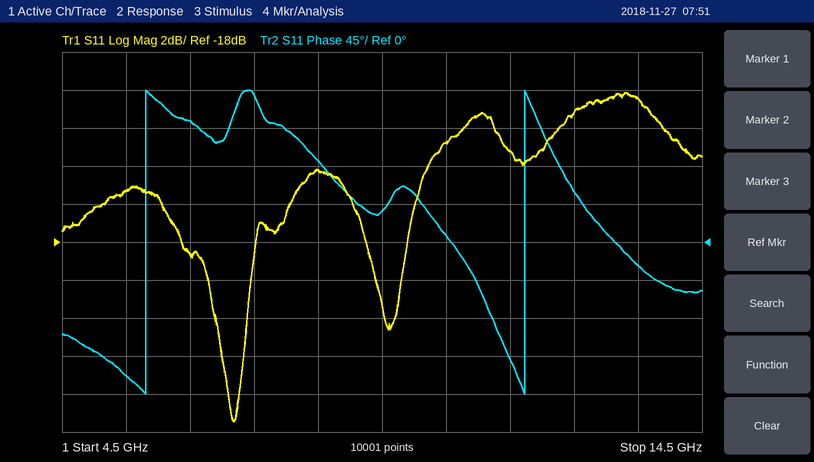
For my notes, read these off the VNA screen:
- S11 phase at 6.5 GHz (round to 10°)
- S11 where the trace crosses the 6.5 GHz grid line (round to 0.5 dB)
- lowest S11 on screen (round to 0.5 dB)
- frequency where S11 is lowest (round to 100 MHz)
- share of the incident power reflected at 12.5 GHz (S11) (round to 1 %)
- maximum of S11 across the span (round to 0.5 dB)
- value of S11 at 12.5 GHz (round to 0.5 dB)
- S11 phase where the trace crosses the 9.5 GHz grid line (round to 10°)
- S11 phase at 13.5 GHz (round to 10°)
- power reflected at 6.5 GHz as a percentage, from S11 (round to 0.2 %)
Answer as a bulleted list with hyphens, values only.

- 140°
- -18.5 dB
- -27.5 dB
- 7.2 GHz
- 8 %
- -10.0 dB
- -11.0 dB
- 40°
- -30°
- 1.4 %
